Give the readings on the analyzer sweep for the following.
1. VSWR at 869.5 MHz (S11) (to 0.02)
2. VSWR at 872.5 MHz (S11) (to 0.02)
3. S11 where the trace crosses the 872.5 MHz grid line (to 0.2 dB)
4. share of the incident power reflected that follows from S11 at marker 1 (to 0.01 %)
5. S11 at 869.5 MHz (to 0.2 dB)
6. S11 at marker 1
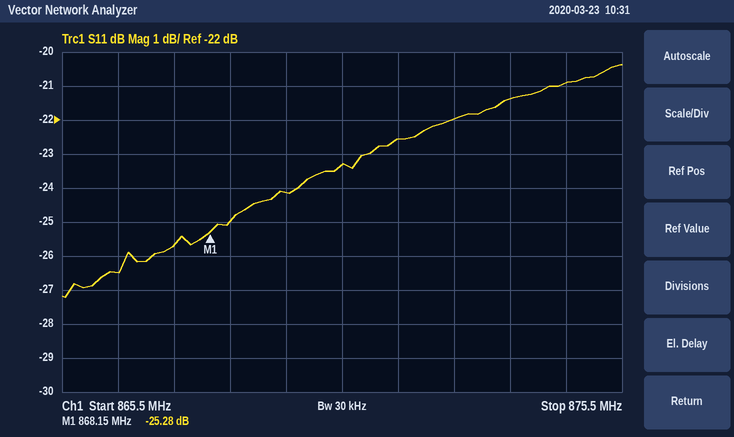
1.14
1.18
-22.0 dB
0.30 %
-24.2 dB
-25.28 dB
